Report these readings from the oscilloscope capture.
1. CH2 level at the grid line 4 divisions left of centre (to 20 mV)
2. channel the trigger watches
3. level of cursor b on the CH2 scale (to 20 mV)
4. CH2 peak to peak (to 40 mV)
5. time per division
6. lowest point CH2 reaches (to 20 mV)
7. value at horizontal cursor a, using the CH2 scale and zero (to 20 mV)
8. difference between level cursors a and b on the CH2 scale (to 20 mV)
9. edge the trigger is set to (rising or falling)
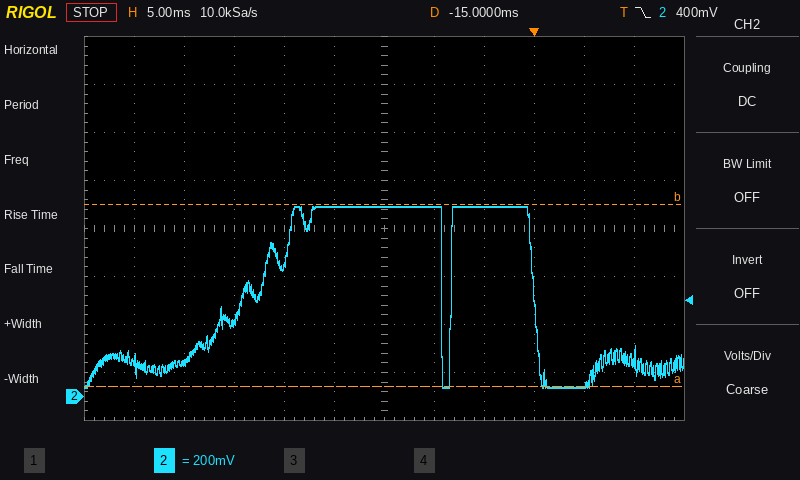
140 mV
CH2
800 mV
760 mV
5 ms
40 mV
40 mV
760 mV
falling
